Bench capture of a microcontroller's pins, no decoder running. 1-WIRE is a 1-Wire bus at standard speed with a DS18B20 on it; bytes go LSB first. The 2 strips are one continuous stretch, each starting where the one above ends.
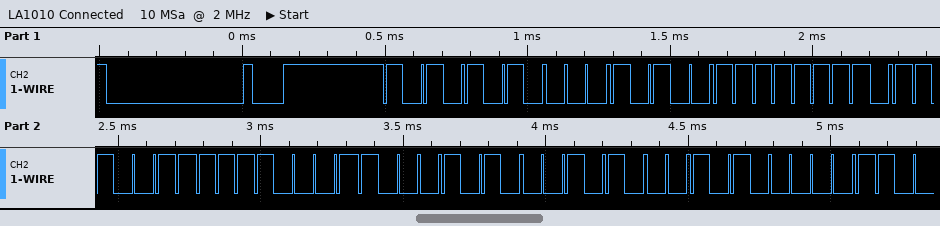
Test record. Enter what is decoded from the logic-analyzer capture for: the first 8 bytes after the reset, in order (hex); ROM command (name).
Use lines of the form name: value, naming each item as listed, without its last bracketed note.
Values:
the first 8 bytes after the reset, in order: 55 28 FF CE 8F 51 14 05
ROM command: Match ROM
